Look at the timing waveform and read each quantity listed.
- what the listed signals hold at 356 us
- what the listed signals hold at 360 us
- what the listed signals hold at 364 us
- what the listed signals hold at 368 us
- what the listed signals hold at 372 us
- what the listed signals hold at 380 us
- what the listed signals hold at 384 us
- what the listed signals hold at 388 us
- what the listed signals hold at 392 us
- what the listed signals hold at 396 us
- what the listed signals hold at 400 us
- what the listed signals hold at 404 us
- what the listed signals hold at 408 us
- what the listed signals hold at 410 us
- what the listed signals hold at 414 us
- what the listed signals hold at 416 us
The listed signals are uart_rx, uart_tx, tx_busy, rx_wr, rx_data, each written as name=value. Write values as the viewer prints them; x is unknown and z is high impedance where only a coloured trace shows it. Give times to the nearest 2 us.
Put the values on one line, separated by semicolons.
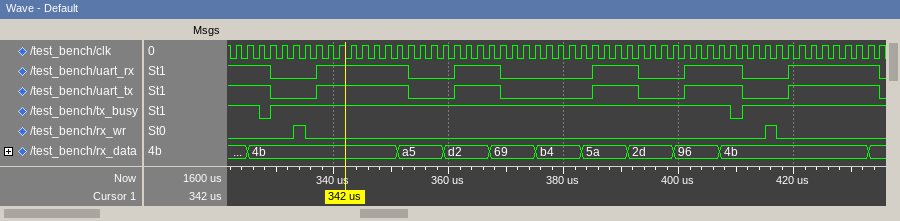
uart_rx=0, uart_tx=0, tx_busy=1, rx_wr=0, rx_data=a5; uart_rx=0, uart_tx=0, tx_busy=1, rx_wr=0, rx_data=d2; uart_rx=1, uart_tx=1, tx_busy=1, rx_wr=0, rx_data=d2; uart_rx=1, uart_tx=1, tx_busy=1, rx_wr=0, rx_data=69; uart_rx=0, uart_tx=0, tx_busy=1, rx_wr=0, rx_data=69; uart_rx=0, uart_tx=0, tx_busy=1, rx_wr=0, rx_data=b4; uart_rx=0, uart_tx=0, tx_busy=1, rx_wr=0, rx_data=5a; uart_rx=1, uart_tx=1, tx_busy=1, rx_wr=0, rx_data=5a; uart_rx=1, uart_tx=1, tx_busy=1, rx_wr=0, rx_data=2d; uart_rx=0, uart_tx=0, tx_busy=1, rx_wr=0, rx_data=2d; uart_rx=0, uart_tx=0, tx_busy=1, rx_wr=0, rx_data=96; uart_rx=1, uart_tx=1, tx_busy=1, rx_wr=0, rx_data=96; uart_rx=1, uart_tx=1, tx_busy=1, rx_wr=0, rx_data=4b; uart_rx=1, uart_tx=1, tx_busy=0, rx_wr=0, rx_data=4b; uart_rx=0, uart_tx=0, tx_busy=1, rx_wr=0, rx_data=4b; uart_rx=0, uart_tx=0, tx_busy=1, rx_wr=1, rx_data=4b
